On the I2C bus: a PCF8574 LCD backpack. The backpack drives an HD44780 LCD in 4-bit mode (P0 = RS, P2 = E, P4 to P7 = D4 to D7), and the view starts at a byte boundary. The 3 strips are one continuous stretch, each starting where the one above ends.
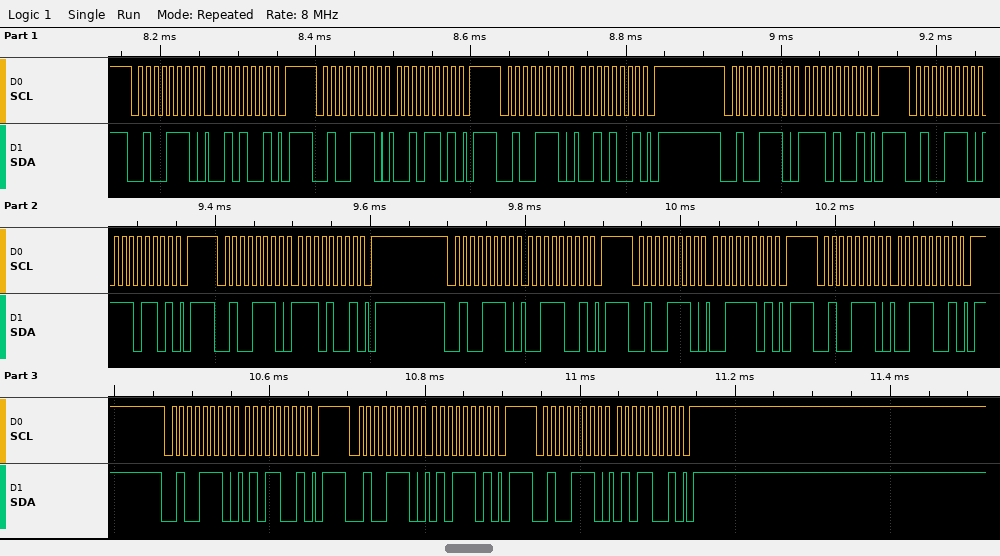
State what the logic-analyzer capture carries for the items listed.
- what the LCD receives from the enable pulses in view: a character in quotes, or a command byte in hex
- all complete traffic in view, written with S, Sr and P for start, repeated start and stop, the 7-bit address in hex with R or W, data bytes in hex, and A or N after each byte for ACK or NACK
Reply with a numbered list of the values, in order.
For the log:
1. '.' '5'
2. S 27W A 29 A P S 27W A 2D A P S 27W A 29 A P S 27W A E9 A P S 27W A ED A P S 27W A E9 A P S 27W A 39 A P S 27W A 3D A P S 27W A 39 A P S 27W A 59 A P S 27W A 5D A P S 27W A 59 A P
